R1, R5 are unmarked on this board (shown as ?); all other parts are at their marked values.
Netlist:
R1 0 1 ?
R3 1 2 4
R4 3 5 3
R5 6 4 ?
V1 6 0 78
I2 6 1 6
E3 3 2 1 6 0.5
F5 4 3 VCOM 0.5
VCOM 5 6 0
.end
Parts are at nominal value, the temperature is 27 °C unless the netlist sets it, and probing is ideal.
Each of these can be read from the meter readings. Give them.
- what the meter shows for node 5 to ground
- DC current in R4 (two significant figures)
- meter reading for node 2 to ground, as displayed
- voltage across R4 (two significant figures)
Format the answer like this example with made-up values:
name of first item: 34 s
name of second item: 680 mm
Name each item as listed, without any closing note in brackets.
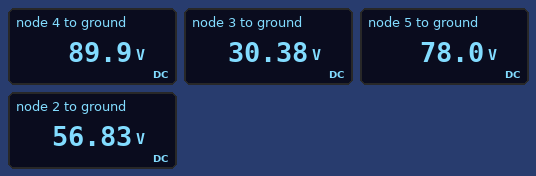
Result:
what the meter shows for node 5 to ground: 78.0 V
DC current in R4: 16 A
meter reading for node 2 to ground, as displayed: 56.83 V
voltage across R4: 48 V
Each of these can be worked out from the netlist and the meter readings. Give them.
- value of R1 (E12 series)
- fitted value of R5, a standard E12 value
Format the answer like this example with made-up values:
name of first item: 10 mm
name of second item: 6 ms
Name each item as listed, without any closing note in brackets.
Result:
value of R1: 1.8 Ω
fitted value of R5, a standard E12 value: 1.5 Ω
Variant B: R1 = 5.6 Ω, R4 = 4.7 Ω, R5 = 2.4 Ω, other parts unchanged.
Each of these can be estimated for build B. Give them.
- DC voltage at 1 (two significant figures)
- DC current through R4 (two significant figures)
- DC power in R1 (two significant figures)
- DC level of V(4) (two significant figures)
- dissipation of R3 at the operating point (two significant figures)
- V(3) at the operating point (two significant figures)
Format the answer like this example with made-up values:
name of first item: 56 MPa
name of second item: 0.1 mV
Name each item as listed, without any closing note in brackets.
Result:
DC voltage at 1: 51 V
DC current through R4: 6.1 A
DC power in R1: 460 W
DC level of V(4): 85 V
dissipation of R3 at the operating point: 37 W
V(3) at the operating point: 49 V
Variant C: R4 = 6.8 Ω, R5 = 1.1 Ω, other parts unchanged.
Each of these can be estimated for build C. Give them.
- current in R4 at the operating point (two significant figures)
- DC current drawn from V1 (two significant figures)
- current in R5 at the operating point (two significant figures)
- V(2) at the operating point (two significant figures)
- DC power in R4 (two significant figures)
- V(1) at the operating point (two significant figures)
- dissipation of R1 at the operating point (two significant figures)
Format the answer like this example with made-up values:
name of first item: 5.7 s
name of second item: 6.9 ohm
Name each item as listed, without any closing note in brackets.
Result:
current in R4 at the operating point: 9.9 A
DC current drawn from V1: 11 A
current in R5 at the operating point: 5.0 A
V(2) at the operating point: 40 V
DC power in R4: 670 W
V(1) at the operating point: 20 V
dissipation of R1 at the operating point: 220 W
